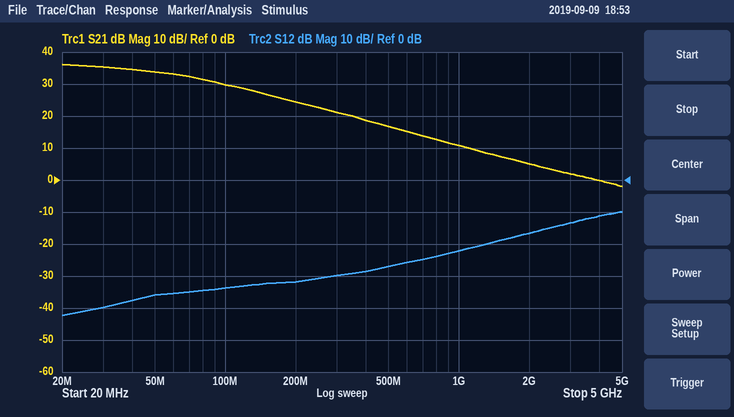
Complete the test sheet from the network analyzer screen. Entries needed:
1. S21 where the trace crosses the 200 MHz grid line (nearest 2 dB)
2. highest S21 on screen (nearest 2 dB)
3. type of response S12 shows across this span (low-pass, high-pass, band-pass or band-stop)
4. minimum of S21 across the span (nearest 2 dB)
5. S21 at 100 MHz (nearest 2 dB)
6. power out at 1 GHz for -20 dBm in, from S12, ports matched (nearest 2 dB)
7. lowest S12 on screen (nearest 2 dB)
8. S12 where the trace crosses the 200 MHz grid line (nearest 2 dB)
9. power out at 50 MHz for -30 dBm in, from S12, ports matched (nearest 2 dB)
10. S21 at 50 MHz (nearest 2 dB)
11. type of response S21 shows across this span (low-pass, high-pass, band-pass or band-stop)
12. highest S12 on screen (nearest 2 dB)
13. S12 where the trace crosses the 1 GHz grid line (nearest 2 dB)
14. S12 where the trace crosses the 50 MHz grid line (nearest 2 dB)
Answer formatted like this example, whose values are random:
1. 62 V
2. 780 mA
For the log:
1. 24 dB
2. 36 dB
3. high-pass
4. -2 dB
5. 30 dB
6. -42 dBm
7. -42 dB
8. -32 dB
9. -66 dBm
10. 34 dB
11. low-pass
12. -10 dB
13. -22 dB
14. -36 dB
